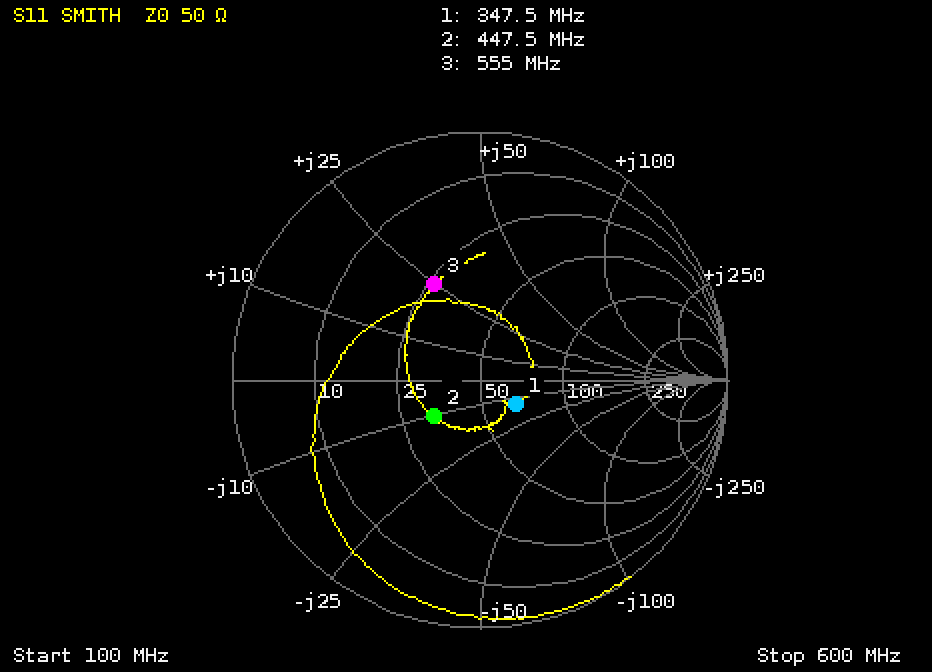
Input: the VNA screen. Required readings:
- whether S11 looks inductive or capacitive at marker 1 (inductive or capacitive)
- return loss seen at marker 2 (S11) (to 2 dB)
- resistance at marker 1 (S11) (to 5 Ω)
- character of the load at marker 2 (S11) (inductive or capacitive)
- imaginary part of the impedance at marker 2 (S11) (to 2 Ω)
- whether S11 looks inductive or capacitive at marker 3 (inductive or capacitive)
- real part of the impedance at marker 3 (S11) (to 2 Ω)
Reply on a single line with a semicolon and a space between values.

capacitive; 12 dB; 65 Ω; capacitive; -10 Ω; inductive; 26 Ω
